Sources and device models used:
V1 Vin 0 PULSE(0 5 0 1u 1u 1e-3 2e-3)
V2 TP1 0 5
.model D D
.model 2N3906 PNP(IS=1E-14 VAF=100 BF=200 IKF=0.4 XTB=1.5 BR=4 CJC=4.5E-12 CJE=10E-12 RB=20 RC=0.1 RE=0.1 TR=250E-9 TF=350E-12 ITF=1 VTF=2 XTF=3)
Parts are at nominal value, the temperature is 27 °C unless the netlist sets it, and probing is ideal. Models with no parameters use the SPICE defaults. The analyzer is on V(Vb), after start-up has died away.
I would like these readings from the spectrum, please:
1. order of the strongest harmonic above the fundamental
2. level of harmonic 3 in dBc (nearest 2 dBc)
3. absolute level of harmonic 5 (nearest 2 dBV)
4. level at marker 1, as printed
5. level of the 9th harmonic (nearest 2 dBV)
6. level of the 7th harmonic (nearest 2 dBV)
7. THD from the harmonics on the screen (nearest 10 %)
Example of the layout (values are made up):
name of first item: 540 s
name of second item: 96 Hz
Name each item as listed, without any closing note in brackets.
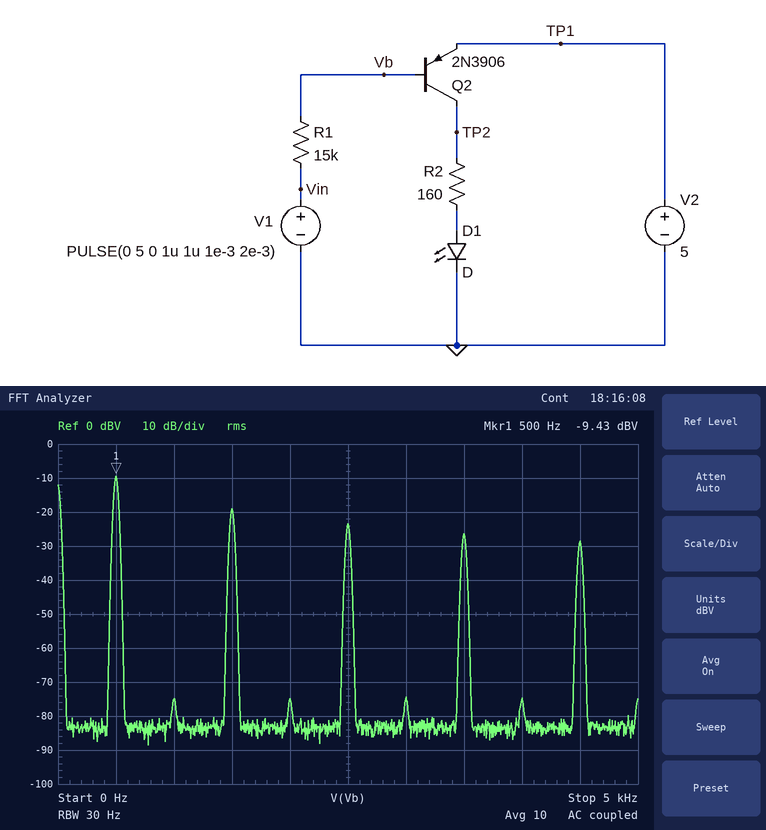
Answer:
order of the strongest harmonic above the fundamental: 3
level of harmonic 3 in dBc: -10 dBc
absolute level of harmonic 5: -24 dBV
level at marker 1, as printed: -9.43 dBV
level of the 9th harmonic: -28 dBV
level of the 7th harmonic: -26 dBV
THD from the harmonics on the screen: 40 %
